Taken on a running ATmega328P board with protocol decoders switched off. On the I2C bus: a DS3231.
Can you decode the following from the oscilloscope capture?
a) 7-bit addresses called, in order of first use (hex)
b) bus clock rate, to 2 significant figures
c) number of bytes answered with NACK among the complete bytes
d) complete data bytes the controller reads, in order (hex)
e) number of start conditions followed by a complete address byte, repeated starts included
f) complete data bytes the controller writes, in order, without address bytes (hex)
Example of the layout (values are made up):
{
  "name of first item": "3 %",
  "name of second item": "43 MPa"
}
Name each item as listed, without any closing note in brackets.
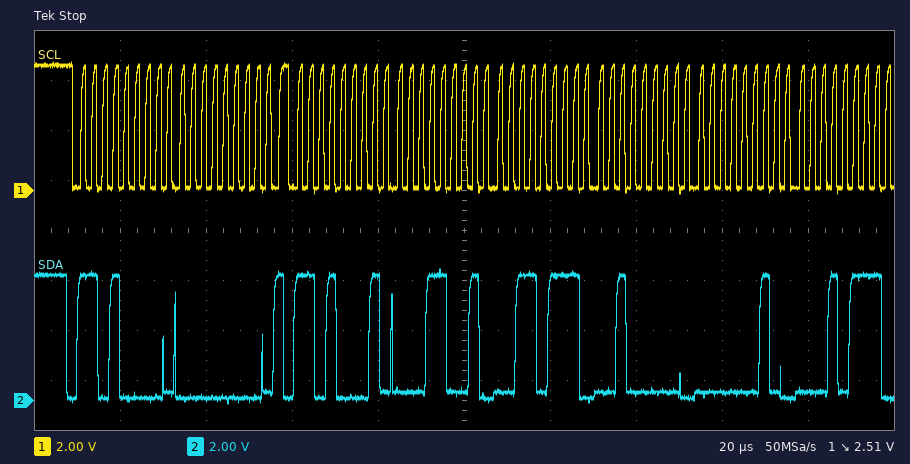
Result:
{
  "7-bit addresses called, in order of first use": "0x68",
  "bus clock rate, to 2 significant figures": "400 kHz",
  "number of bytes answered with NACK among the complete bytes": "0",
  "complete data bytes the controller reads, in order": "19 37 20 02 17",
  "number of start conditions followed by a complete address byte, repeated starts included": "2",
  "complete data bytes the controller writes, in order, without address bytes": "00"
}
